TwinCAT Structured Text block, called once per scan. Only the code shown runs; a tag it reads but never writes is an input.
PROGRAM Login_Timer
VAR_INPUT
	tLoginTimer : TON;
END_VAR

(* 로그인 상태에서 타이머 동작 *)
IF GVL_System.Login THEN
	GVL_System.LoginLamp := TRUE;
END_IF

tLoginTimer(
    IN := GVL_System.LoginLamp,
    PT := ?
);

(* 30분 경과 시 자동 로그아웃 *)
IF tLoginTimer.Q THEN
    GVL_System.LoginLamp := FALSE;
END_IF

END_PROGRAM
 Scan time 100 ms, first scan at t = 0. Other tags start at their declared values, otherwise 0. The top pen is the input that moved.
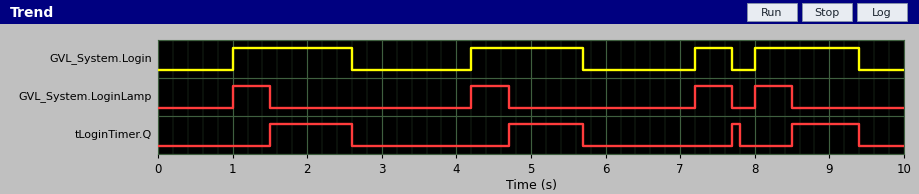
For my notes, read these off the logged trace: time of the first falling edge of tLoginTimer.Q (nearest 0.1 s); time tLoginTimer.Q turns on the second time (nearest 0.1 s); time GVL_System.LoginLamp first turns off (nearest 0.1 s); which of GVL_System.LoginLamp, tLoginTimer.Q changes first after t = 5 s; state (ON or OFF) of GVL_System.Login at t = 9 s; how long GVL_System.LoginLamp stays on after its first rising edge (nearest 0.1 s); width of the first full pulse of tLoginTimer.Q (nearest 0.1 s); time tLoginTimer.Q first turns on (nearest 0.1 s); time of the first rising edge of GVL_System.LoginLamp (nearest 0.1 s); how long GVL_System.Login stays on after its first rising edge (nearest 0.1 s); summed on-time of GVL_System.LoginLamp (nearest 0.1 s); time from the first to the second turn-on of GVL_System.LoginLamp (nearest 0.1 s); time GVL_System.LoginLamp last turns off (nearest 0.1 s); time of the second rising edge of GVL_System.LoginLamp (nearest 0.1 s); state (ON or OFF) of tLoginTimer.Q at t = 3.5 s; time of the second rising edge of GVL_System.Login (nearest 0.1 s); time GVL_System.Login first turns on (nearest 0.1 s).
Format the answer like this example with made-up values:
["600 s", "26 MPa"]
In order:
["2.6 s", "4.7 s", "1.5 s", "tLoginTimer.Q", "ON", "0.5 s", "1.1 s", "1.5 s", "1.0 s", "1.6 s", "2.0 s", "3.2 s", "8.5 s", "4.2 s", "OFF", "4.2 s", "1.0 s"]
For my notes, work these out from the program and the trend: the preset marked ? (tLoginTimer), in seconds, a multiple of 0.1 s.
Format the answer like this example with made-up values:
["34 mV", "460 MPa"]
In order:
["0.5 s"]
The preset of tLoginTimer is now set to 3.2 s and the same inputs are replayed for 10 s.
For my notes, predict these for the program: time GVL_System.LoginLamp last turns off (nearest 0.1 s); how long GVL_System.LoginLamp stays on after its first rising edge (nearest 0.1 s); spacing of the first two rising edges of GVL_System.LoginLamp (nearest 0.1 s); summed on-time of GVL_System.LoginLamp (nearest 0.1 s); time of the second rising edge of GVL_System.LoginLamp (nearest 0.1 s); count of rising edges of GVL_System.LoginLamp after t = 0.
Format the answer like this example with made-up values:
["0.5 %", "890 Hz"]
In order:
["4.2 s", "3.2 s", "6.2 s", "6.0 s", "7.2 s", "2"]
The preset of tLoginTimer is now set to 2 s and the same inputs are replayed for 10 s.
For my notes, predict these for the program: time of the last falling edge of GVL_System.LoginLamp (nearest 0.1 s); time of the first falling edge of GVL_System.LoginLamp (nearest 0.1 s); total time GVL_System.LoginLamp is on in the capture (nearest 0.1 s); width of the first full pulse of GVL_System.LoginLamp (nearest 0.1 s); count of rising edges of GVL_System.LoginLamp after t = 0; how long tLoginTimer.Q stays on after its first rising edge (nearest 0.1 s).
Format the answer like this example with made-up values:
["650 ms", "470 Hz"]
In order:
["9.2 s", "3.0 s", "6.0 s", "2.0 s", "3", "0.1 s"]
